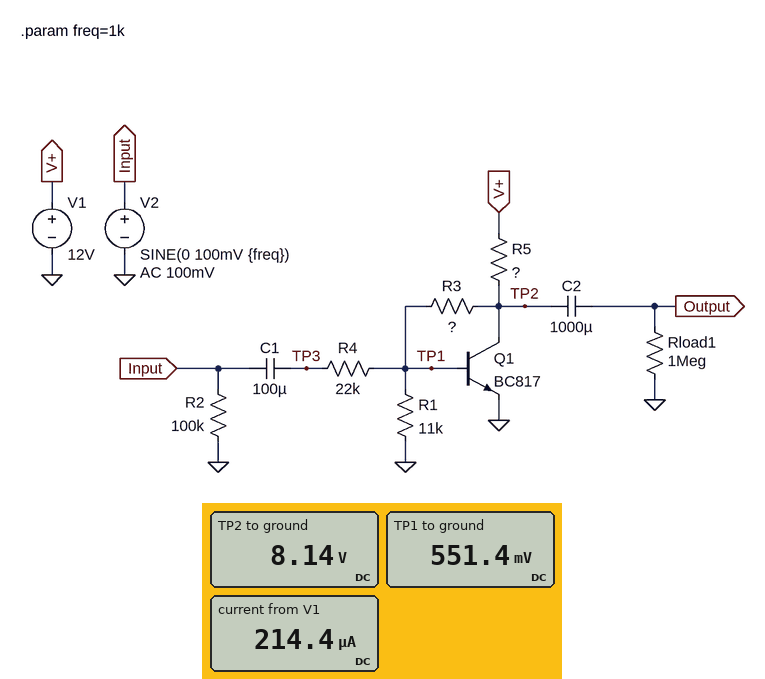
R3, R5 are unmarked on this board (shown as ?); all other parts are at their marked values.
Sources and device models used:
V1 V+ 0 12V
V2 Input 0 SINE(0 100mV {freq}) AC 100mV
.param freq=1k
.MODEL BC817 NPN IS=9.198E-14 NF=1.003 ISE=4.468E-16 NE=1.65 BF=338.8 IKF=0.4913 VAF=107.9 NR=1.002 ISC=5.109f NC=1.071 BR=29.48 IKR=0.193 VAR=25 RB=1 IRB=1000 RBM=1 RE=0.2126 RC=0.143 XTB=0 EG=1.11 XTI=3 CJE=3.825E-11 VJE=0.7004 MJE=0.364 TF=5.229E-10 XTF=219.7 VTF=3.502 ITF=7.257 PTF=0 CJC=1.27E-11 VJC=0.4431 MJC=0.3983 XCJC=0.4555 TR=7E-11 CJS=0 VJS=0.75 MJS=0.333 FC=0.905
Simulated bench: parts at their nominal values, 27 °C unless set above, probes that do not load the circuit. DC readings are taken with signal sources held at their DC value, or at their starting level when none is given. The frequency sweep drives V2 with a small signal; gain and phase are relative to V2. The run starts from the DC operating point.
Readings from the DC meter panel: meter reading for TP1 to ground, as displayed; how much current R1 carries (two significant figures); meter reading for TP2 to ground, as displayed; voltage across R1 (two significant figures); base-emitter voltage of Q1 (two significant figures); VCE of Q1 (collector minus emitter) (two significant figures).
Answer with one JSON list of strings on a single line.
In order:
["551.4 mV", "50 µA", "8.14 V", "550 mV", "550 mV", "8.1 V"]
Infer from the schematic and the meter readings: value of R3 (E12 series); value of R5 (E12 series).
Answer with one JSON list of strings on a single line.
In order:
["150 kΩ", "18 kΩ"]
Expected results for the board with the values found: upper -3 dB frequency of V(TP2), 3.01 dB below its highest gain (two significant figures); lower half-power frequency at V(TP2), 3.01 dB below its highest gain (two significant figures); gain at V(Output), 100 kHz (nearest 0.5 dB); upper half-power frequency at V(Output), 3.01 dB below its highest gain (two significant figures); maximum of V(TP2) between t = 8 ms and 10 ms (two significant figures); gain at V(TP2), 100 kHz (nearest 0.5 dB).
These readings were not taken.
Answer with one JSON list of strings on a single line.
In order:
["280 kHz", "68 mHz", "14.0 dB", "280 kHz", "8.7 V", "14.0 dB"]
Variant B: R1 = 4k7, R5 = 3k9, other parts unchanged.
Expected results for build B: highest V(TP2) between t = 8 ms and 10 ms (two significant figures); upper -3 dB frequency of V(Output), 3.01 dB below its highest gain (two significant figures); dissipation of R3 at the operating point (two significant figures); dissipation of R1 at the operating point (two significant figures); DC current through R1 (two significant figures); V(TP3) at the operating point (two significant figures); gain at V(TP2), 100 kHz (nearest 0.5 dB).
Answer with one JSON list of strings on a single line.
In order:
["12 V", "15 MHz", "860 µW", "27 µW", "76 µA", "360 mV", "-52.0 dB"]
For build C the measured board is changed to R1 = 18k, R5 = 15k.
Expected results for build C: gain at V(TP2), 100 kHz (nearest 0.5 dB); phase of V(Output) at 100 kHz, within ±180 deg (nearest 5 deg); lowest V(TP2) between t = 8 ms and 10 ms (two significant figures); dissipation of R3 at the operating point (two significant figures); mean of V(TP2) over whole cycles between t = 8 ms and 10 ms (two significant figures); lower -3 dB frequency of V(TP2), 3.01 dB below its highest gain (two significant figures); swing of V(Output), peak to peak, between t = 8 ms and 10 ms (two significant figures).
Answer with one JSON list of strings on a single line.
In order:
["15.0 dB", "155 deg", "4.9 V", "160 µW", "5.5 V", "70 mHz", "1.2 V"]
